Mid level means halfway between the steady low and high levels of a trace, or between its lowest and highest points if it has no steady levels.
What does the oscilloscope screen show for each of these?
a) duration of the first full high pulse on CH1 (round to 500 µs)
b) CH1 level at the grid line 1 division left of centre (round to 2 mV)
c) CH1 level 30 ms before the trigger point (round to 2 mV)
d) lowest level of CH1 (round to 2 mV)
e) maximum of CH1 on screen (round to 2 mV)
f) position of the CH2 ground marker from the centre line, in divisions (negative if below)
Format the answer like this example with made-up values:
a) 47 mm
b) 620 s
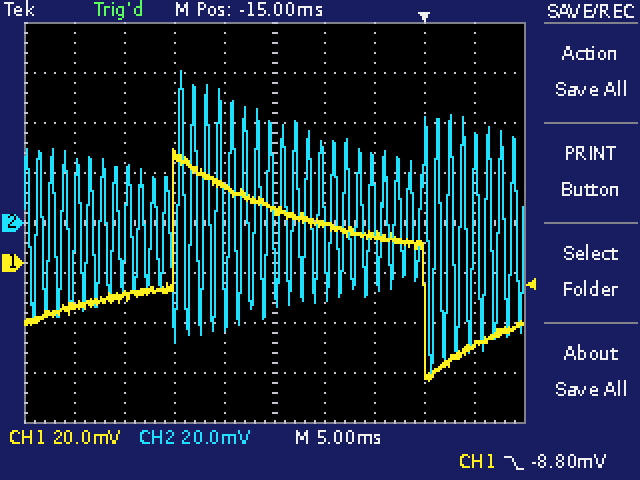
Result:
a) 25.0 ms
b) 32 mV
c) -14 mV
d) -48 mV
e) 46 mV
f) 0.0 div
